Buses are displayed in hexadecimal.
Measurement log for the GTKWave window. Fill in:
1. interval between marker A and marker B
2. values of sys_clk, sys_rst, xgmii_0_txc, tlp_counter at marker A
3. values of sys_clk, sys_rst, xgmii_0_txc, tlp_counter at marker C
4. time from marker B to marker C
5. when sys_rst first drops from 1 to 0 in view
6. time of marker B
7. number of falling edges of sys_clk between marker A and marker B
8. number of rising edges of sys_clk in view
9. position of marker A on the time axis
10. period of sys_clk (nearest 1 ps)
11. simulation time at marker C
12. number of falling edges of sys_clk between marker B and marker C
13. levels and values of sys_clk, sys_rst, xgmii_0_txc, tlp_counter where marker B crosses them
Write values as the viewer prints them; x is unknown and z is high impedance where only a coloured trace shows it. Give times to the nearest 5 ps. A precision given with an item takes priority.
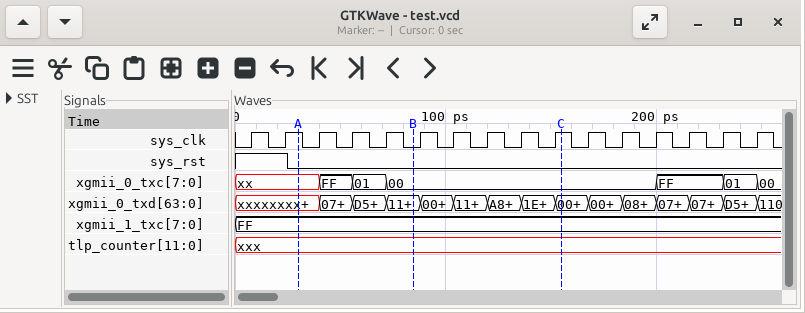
55 ps
sys_clk=1, sys_rst=0, xgmii_0_txc=xx, tlp_counter=xxx
sys_clk=1, sys_rst=0, xgmii_0_txc=00, tlp_counter=xxx
70 ps
25 ps
85 ps
4
16
30 ps
16 ps
155 ps
4
sys_clk=0, sys_rst=0, xgmii_0_txc=00, tlp_counter=xxx
